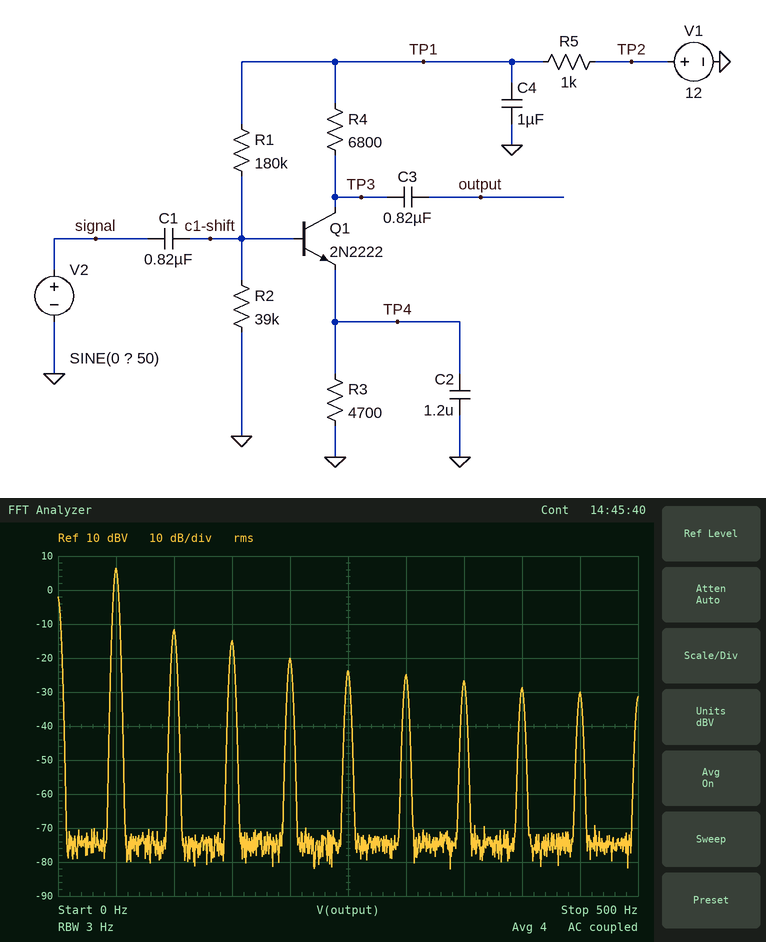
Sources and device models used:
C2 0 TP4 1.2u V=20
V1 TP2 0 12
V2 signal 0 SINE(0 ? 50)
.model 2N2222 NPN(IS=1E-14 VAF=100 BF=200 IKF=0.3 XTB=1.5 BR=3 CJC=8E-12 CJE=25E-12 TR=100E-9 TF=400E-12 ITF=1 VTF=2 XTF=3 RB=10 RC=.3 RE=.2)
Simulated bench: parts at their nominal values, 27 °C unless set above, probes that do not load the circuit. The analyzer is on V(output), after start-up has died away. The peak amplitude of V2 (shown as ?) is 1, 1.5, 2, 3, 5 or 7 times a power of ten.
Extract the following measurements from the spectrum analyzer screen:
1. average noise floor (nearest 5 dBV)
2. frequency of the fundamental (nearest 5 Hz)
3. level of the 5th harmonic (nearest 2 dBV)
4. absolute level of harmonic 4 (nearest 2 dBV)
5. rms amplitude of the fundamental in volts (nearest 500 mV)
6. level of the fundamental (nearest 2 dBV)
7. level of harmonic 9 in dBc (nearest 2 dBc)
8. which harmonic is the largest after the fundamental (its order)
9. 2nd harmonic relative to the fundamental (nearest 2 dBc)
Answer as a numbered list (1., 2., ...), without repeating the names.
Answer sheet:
1. -75 dBV
2. 50 Hz
3. -24 dBV
4. -20 dBV
5. 2.0 V
6. 6 dBV
7. -36 dBc
8. 2
9. -18 dBc
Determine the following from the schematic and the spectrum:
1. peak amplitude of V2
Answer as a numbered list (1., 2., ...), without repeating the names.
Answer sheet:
1. 1 V
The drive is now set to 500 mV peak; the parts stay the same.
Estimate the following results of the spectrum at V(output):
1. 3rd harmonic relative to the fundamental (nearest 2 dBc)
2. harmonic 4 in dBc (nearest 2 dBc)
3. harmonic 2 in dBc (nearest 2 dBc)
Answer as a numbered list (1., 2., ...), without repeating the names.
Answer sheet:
1. -46 dBc
2. -54 dBc
3. -36 dBc
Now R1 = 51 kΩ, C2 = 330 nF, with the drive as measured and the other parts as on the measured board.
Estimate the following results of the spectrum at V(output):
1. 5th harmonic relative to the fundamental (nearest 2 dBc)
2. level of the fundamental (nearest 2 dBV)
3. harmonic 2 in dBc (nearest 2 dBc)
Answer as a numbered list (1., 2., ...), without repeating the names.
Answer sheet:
1. -38 dBc
2. 0 dBV
3. -16 dBc
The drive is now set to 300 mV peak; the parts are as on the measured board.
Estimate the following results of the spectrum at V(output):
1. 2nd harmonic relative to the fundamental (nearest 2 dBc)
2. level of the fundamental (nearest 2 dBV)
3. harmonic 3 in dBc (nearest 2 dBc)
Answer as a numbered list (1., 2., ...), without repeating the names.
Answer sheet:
1. -42 dBc
2. -4 dBV
3. -56 dBc
